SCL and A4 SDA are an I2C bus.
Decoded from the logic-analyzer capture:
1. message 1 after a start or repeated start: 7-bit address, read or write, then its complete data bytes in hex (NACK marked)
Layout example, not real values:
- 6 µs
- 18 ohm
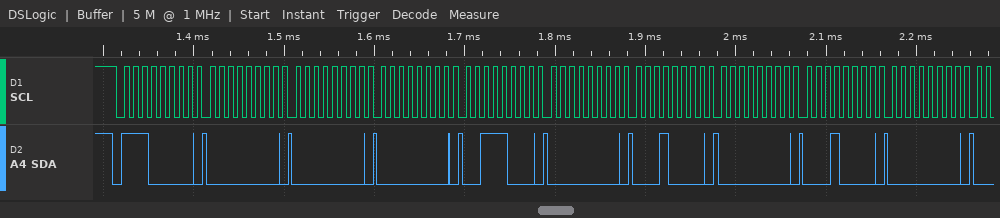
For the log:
- 0x70 write: 00 00 00 38 00 10 00 10 00
